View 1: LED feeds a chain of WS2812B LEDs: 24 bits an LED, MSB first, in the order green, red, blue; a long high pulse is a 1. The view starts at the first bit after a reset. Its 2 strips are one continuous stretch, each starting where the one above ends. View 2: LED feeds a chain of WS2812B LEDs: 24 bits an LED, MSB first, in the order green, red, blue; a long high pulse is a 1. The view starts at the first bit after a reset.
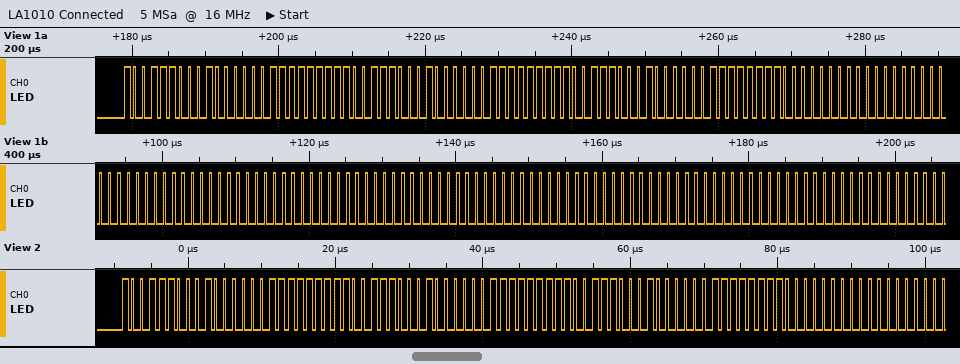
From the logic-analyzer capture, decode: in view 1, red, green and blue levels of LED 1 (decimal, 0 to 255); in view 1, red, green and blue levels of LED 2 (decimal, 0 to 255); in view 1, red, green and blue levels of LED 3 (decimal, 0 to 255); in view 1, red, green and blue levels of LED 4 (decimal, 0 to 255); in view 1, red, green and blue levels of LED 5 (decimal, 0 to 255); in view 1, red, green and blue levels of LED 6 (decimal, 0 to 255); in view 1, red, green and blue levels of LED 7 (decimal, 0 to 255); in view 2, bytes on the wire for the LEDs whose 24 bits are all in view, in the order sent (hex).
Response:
64, 156, 255
64, 156, 255
64, 156, 255
0, 0, 0
0, 0, 0
0, 0, 0
0, 0, 0
9C 40 FF 9C 40 FF 9C 40 FF
